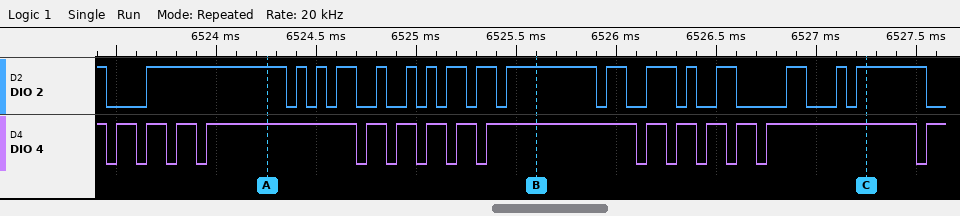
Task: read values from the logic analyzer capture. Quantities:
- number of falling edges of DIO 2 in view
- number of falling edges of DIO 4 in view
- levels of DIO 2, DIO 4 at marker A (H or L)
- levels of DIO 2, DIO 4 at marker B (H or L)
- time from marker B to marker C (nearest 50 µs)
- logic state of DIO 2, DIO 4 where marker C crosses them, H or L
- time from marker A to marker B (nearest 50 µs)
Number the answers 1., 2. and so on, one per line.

1. 18
2. 15
3. DIO 2=H, DIO 4=H
4. DIO 2=H, DIO 4=H
5. 1650 µs
6. DIO 2=H, DIO 4=H
7. 1350 µs
